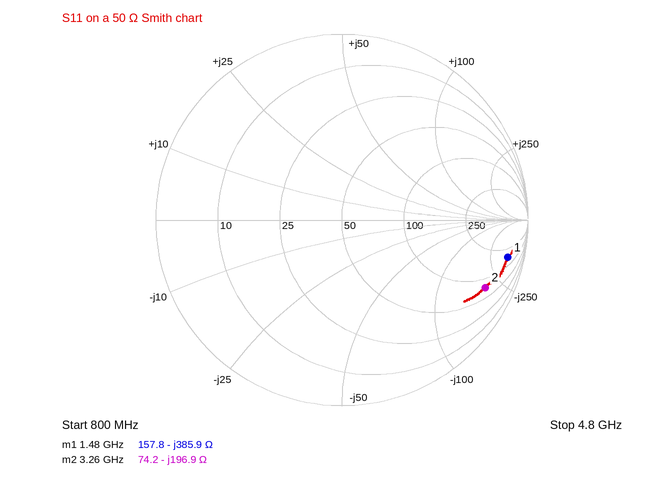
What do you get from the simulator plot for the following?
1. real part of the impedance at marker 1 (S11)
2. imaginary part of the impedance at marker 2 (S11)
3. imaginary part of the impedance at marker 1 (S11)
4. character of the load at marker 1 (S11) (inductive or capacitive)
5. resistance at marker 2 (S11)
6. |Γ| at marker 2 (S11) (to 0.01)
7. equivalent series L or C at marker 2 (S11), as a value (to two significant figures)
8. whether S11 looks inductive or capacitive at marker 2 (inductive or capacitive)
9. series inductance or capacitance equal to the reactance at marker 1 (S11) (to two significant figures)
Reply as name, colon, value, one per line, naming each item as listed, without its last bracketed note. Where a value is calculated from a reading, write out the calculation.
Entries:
real part of the impedance at marker 1: 157.8 Ω
imaginary part of the impedance at marker 2: -196.9 Ω
imaginary part of the impedance at marker 1: -385.9 Ω
character of the load at marker 1 (S11): capacitive
resistance at marker 2: 74.2 Ω
|Γ| at marker 2 (S11): 0.85
equivalent series L or C at marker 2 (S11), as a value: C = 1/(2π × 3.26 GHz × 196.9 Ω) ≈ 248 fF, so 250 fF to two significant figures
whether S11 looks inductive or capacitive at marker 2: capacitive
series inductance or capacitance equal to the reactance at marker 1 (S11): C = 1/(2π × 1.48 GHz × 385.9 Ω) ≈ 279 fF, so 280 fF to two significant figures
